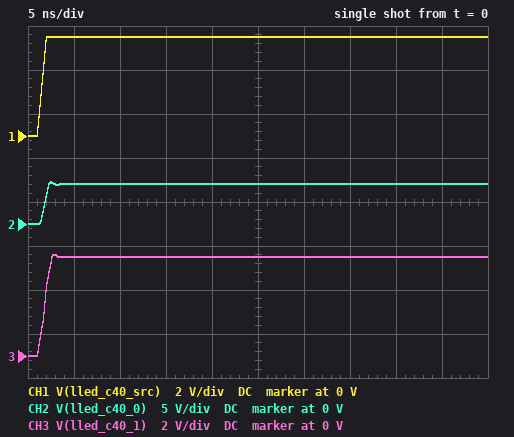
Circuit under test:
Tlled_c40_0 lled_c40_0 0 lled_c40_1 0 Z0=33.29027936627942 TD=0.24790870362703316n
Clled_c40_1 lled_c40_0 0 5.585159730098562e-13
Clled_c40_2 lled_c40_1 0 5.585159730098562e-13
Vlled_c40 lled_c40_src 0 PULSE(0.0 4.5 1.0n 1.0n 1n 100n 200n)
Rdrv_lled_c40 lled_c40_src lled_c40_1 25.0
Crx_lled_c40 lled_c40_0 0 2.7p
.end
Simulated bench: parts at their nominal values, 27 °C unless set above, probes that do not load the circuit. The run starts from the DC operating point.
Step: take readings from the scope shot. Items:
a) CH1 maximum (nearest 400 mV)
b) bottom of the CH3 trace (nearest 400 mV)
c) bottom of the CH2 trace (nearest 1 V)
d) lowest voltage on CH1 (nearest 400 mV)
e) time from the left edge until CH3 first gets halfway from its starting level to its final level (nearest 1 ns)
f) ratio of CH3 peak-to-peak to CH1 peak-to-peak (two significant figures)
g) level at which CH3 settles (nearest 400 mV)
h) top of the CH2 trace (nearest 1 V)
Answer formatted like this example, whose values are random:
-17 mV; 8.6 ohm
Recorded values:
4.4 V; 0 V; 0 V; 0 V; 2 ns; 1.0; 4.4 V; 5 V
